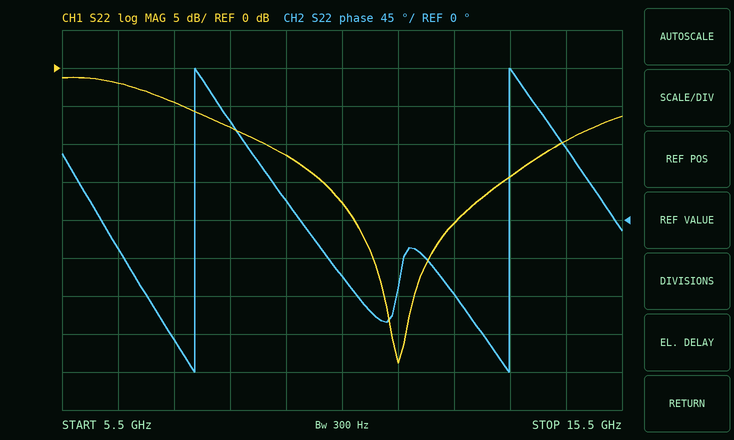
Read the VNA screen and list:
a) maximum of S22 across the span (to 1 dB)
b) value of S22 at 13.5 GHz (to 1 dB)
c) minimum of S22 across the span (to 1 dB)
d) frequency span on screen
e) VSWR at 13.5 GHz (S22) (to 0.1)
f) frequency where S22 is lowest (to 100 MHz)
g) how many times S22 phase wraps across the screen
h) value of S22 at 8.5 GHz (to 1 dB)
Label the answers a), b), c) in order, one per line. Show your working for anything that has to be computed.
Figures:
a) -1 dB
b) -14 dB
c) -39 dB
d) 10 GHz
e) |Γ| = 10^(-14/20) = 0.1995; VSWR = (1 + 0.1995)/(1 − 0.1995) ≈ 1.5
f) 11.5 GHz
g) 2
h) -8 dB
